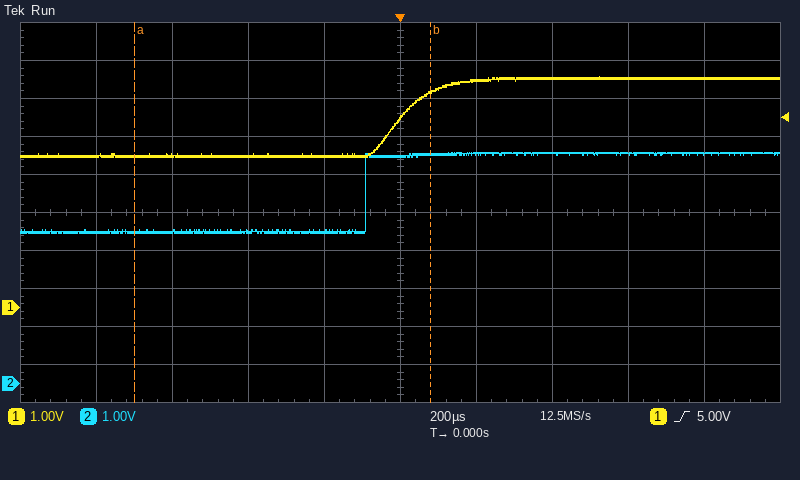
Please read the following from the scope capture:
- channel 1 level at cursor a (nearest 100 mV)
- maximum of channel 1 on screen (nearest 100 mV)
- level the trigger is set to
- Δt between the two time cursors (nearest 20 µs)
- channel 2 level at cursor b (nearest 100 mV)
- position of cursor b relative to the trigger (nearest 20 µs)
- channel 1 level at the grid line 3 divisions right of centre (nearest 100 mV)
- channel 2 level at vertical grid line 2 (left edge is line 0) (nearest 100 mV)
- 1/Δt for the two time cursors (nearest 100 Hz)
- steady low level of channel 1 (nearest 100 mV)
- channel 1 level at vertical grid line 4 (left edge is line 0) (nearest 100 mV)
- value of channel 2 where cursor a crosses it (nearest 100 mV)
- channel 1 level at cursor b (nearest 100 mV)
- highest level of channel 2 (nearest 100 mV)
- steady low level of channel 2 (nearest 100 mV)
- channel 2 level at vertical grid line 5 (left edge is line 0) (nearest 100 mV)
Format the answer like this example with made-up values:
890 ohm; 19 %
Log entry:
4.0 V; 6.1 V; 5.00 V; 780 µs; 6.0 V; +80 µs; 6.0 V; 4.0 V; 1.3 kHz; 4.0 V; 4.0 V; 4.0 V; 5.7 V; 6.1 V; 4.0 V; 6.0 V
